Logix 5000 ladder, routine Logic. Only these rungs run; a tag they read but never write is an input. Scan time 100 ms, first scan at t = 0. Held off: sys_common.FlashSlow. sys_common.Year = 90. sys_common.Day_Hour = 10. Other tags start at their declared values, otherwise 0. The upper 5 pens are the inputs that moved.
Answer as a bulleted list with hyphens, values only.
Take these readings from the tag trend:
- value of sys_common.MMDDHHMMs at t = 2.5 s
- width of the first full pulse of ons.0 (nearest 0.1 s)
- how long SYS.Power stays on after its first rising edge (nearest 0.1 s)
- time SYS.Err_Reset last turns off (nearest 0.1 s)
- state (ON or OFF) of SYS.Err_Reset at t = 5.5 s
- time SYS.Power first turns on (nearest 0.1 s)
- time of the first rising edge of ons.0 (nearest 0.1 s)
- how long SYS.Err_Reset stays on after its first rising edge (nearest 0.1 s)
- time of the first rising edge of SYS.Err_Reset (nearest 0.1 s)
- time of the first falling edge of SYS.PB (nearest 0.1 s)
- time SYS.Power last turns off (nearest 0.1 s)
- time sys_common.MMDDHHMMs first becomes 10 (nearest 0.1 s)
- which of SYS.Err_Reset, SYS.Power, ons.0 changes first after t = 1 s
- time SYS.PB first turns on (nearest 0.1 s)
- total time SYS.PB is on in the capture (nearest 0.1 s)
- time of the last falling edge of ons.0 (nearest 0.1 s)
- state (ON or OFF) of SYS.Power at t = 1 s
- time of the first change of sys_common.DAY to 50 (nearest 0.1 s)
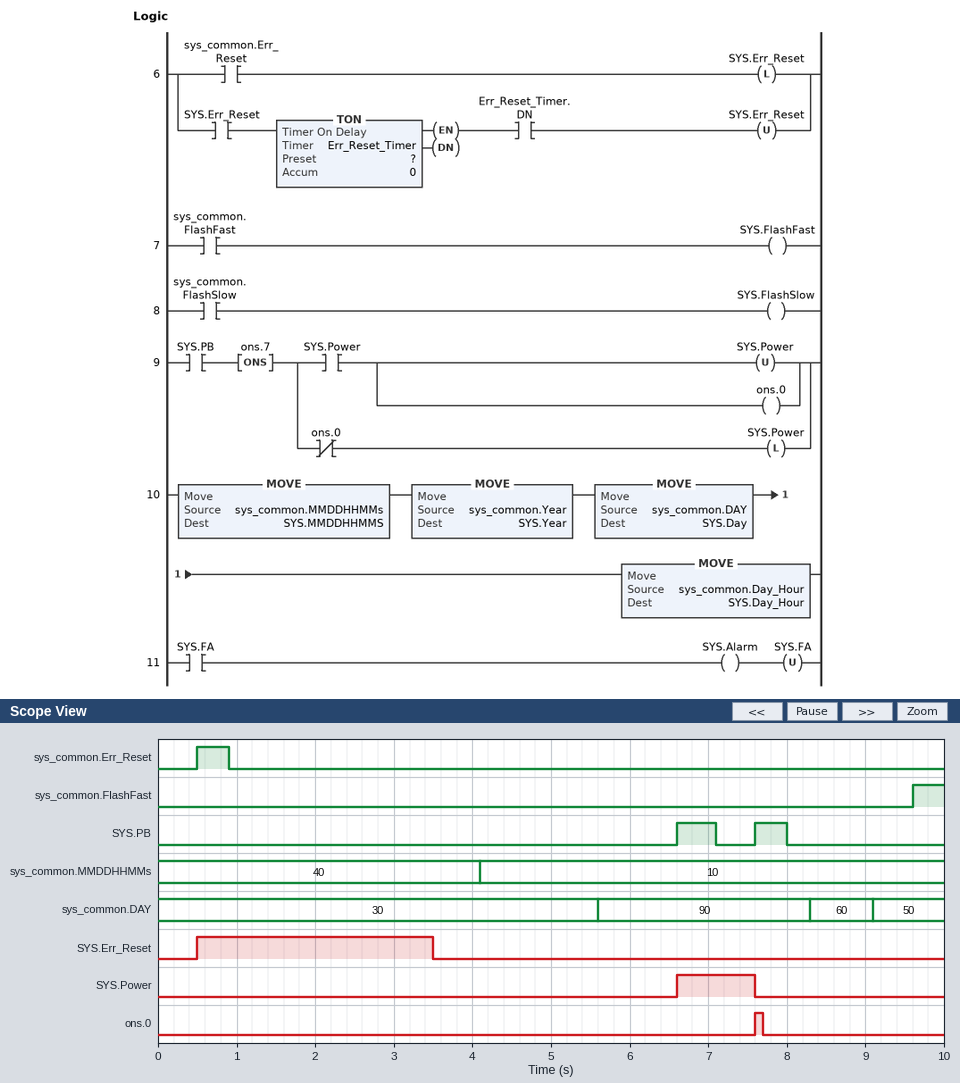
- 40
- 0.1 s
- 1.0 s
- 3.5 s
- OFF
- 6.6 s
- 7.6 s
- 3.0 s
- 0.5 s
- 7.1 s
- 7.6 s
- 4.1 s
- SYS.Err_Reset
- 6.6 s
- 0.9 s
- 7.7 s
- OFF
- 9.1 s
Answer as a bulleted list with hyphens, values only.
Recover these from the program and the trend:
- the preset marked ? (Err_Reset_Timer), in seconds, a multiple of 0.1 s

- 3.0 s
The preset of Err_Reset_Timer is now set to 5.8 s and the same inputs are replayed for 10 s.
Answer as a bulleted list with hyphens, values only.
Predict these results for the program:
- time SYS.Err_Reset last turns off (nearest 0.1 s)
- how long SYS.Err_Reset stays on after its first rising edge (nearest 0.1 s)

- 6.3 s
- 5.8 s
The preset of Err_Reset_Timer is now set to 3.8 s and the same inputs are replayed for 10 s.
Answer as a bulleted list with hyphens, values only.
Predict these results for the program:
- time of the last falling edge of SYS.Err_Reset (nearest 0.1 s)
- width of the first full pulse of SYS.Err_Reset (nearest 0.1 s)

- 4.3 s
- 3.8 s
